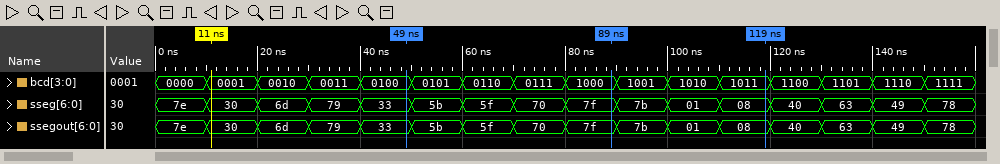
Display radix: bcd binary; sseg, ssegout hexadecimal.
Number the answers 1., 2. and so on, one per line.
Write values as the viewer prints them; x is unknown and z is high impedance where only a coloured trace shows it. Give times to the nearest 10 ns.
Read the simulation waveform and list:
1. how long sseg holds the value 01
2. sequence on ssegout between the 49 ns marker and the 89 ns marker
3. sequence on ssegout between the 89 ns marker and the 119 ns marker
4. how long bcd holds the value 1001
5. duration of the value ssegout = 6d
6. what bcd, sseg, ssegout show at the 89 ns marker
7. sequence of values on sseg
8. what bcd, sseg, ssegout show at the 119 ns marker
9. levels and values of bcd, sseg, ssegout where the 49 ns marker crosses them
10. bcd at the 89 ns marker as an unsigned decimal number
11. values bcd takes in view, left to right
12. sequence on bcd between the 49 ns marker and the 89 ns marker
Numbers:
1. 10 ns
2. 33, 5b, 5f, 70, 7f
3. 7f, 7b, 01, 08
4. 10 ns
5. 10 ns
6. bcd=1000, sseg=7f, ssegout=7f
7. 7e, 30, 6d, 79, 33, 5b, 5f, 70, 7f, 7b, 01, 08, 40, 63, 49, 78
8. bcd=1011, sseg=08, ssegout=08
9. bcd=0100, sseg=33, ssegout=33
10. 8
11. 0000, 0001, 0010, 0011, 0100, 0101, 0110, 0111, 1000, 1001, 1010, 1011, 1100, 1101, 1110, 1111
12. 0100, 0101, 0110, 0111, 1000
